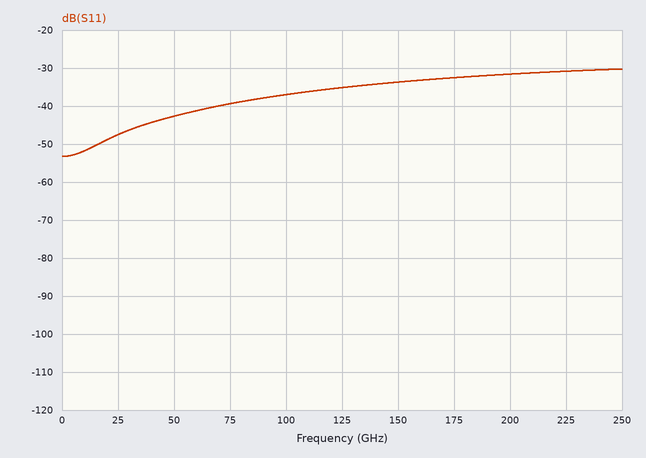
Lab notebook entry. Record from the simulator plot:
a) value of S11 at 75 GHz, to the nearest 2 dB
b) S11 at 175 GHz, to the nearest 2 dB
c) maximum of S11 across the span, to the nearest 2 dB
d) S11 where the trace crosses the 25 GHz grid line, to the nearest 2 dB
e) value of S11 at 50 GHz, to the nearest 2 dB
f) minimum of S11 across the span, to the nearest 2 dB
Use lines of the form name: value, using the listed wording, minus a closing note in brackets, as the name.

value of S11 at 75 GHz, to the nearest 2 dB: -40 dB
S11 at 175 GHz, to the nearest 2 dB: -32 dB
maximum of S11 across the span, to the nearest 2 dB: -30 dB
S11 where the trace crosses the 25 GHz grid line, to the nearest 2 dB: -48 dB
value of S11 at 50 GHz, to the nearest 2 dB: -42 dB
minimum of S11 across the span, to the nearest 2 dB: -54 dB
